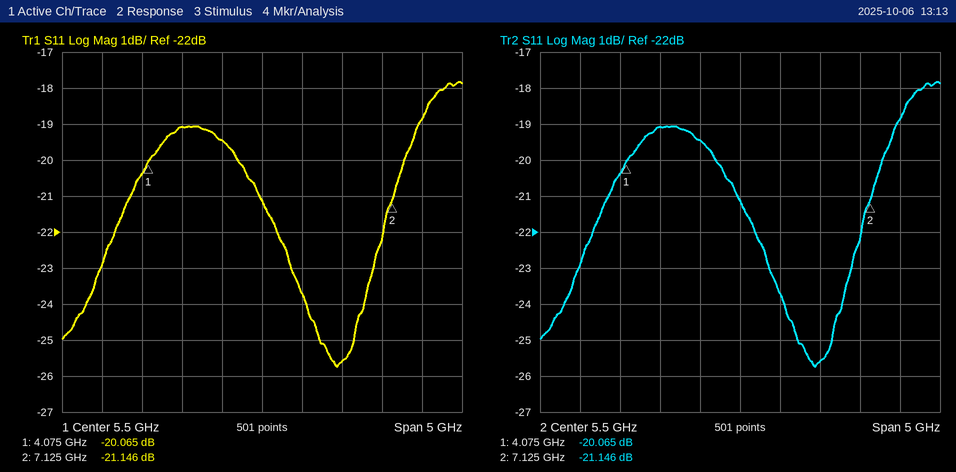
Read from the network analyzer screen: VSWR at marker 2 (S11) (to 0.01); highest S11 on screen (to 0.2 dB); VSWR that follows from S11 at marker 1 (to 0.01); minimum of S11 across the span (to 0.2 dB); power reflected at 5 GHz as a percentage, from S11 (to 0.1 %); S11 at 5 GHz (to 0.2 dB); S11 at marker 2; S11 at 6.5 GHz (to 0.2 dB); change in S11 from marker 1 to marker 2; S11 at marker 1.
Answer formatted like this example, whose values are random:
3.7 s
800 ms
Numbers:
1.19
-17.8 dB
1.22
-25.8 dB
1.1 %
-19.4 dB
-21.146 dB
-25.6 dB
-1.081 dB
-20.065 dB
